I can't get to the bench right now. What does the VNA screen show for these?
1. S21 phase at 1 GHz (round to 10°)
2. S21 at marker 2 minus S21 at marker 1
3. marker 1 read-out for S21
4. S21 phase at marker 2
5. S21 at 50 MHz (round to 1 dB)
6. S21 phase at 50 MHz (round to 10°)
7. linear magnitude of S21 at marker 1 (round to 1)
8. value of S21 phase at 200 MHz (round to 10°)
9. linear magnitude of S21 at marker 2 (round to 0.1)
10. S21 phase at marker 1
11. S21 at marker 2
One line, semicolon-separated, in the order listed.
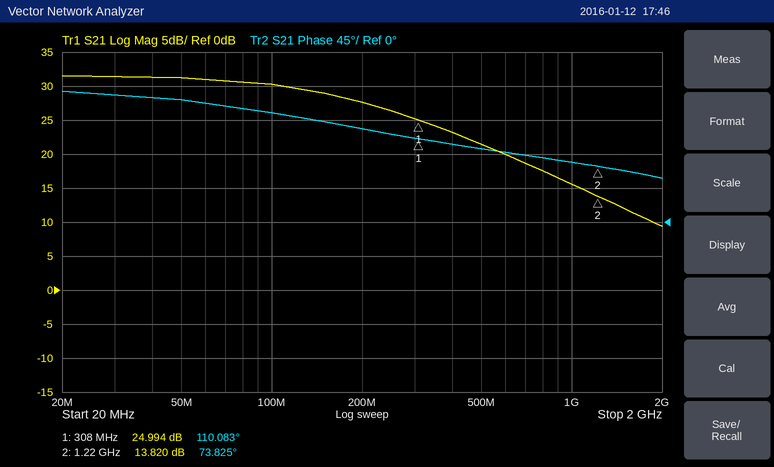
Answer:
80°; -11.174 dB; 24.994 dB; 73.825°; 31 dB; 160°; 18; 120°; 4.9; 110.083°; 13.820 dB
